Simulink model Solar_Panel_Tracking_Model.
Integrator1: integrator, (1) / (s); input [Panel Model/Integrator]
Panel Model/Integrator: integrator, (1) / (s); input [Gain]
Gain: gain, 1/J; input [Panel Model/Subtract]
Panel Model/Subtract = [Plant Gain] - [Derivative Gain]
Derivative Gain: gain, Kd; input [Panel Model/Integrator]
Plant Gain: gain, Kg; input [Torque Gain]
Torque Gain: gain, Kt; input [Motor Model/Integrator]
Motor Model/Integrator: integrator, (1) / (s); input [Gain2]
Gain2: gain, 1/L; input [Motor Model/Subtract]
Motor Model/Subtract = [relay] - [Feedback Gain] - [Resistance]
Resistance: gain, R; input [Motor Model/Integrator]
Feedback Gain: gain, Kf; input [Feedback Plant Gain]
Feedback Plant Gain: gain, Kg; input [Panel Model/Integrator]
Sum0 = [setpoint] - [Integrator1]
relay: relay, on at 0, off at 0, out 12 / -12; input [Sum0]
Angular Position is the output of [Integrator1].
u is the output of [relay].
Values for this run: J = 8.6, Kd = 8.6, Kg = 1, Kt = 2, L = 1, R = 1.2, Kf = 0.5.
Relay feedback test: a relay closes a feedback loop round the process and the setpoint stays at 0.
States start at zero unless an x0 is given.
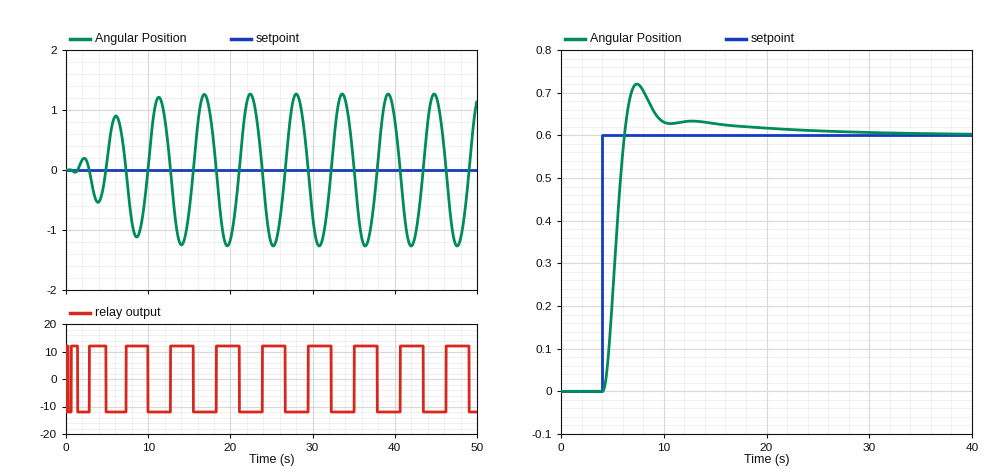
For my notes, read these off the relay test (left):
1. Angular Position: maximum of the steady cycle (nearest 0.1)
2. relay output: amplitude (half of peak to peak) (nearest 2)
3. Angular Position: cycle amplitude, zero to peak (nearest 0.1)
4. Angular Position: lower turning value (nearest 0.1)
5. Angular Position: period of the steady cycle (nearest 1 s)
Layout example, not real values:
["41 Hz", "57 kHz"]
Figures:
["1.3", "12", "1.3", "-1.3", "6 s"]
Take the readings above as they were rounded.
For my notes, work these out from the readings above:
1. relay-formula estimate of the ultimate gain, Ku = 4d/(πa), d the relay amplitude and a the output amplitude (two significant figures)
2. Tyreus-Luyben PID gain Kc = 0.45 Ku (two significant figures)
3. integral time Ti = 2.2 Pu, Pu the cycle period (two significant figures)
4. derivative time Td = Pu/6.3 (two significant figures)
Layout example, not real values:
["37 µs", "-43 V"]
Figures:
["12", "5.4", "13 s", "0.95 s"]
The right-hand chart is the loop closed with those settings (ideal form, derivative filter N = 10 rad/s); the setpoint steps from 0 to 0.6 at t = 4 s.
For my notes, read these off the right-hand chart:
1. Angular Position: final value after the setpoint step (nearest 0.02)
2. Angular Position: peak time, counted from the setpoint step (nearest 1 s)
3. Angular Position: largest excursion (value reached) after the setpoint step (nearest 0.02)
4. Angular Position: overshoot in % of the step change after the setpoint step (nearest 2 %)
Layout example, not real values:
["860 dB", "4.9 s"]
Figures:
["0.60", "3 s", "0.72", "20 %"]
